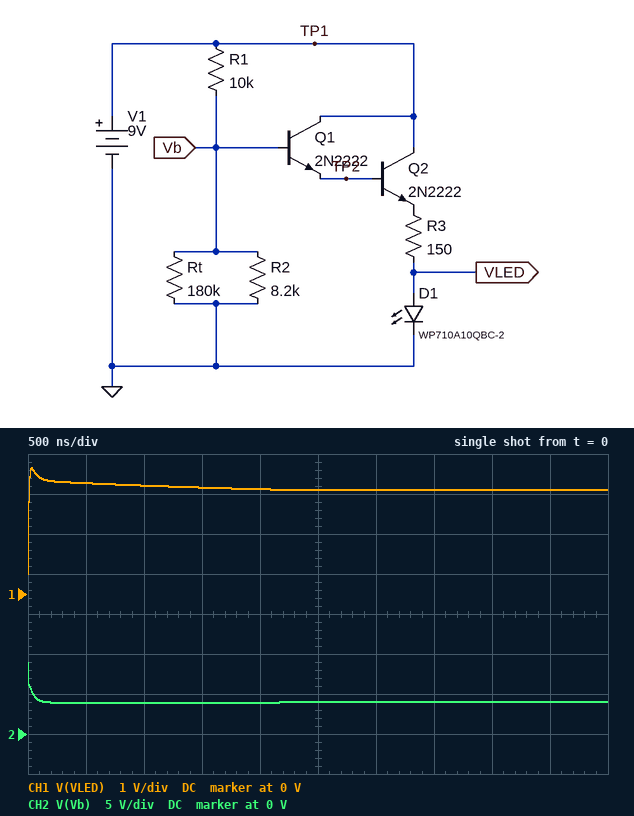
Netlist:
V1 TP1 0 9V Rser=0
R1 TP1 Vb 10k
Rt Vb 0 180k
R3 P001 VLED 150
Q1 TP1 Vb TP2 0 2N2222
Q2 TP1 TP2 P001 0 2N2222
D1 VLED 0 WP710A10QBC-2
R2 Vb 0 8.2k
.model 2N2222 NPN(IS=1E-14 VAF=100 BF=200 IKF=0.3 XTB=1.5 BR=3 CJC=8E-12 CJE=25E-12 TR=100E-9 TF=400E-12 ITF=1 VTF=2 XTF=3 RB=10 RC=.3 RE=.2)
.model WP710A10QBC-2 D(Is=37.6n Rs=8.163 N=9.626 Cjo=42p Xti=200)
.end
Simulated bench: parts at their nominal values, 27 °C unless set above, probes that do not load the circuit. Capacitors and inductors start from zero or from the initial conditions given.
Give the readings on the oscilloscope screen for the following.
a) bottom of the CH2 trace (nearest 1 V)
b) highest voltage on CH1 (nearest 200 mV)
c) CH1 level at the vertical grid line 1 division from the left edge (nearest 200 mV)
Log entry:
4 V
3.2 V
2.8 V
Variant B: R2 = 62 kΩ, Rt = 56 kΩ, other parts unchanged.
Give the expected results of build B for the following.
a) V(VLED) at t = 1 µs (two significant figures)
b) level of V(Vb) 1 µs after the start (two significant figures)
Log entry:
3.3 V
6.7 V
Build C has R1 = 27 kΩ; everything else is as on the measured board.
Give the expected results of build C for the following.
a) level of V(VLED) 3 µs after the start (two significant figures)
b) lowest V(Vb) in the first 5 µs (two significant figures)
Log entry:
1.9 V
2.0 V
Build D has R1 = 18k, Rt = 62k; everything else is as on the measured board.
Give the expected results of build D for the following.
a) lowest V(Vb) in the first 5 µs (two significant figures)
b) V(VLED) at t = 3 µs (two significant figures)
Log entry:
2.6 V
2.2 V
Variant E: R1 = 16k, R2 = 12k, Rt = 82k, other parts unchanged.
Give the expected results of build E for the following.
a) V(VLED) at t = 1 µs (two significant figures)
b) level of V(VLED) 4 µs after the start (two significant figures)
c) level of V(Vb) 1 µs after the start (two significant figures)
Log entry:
2.6 V
2.4 V
3.5 V
